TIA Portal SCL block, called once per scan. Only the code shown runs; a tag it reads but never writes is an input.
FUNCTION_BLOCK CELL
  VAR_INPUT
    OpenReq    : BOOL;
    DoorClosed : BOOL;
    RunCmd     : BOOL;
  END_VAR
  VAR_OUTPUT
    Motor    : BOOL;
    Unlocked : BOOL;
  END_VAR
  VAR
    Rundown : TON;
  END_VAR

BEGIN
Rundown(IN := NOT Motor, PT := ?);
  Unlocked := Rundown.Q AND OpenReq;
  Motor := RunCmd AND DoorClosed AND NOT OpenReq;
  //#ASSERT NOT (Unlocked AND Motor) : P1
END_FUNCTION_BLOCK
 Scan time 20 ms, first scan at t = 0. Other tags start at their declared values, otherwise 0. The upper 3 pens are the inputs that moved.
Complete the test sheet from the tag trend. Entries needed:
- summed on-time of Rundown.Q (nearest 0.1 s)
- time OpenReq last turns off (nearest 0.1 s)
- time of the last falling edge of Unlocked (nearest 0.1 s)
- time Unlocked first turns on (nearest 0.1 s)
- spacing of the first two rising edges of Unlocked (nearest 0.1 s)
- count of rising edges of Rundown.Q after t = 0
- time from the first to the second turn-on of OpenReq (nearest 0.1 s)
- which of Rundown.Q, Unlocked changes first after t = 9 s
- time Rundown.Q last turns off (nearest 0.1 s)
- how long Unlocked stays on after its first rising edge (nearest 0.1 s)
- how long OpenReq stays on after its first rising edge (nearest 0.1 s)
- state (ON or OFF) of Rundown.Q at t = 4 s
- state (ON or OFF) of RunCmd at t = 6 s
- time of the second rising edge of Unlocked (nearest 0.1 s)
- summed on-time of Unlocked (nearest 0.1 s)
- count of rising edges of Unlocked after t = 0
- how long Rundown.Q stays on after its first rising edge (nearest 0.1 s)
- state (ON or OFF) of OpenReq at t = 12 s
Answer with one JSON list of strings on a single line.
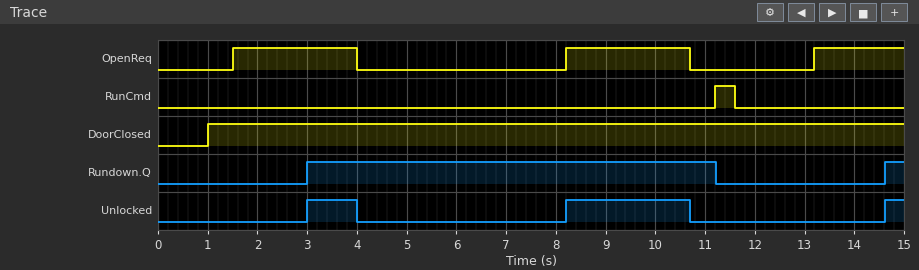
["8.6 s", "10.7 s", "10.7 s", "3.0 s", "5.2 s", "2", "6.7 s", "Unlocked", "11.2 s", "1.0 s", "2.5 s", "ON", "OFF", "8.2 s", "3.9 s", "3", "8.2 s", "OFF"]
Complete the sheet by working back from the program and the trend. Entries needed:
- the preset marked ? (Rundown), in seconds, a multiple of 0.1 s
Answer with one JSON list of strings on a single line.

["3.0 s"]
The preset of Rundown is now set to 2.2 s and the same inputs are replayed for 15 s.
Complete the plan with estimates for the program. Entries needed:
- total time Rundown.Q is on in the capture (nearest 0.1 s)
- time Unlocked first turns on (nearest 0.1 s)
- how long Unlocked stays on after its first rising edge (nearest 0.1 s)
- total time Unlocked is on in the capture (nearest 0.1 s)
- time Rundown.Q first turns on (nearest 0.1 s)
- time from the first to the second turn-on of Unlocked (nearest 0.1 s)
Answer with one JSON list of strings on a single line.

["10.2 s", "2.2 s", "1.8 s", "5.5 s", "2.2 s", "6.0 s"]
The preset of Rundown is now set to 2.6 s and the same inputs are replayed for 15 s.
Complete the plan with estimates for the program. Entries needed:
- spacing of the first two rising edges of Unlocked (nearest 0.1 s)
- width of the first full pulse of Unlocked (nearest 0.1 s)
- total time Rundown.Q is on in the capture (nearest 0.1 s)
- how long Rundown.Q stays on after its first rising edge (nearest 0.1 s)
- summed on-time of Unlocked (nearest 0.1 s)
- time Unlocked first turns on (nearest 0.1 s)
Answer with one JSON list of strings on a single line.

["5.6 s", "1.4 s", "9.4 s", "8.6 s", "4.7 s", "2.6 s"]
